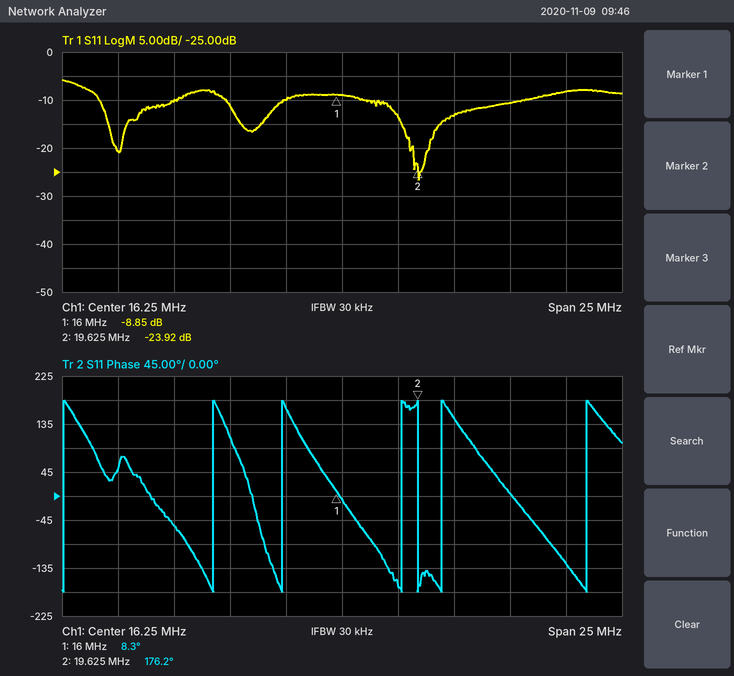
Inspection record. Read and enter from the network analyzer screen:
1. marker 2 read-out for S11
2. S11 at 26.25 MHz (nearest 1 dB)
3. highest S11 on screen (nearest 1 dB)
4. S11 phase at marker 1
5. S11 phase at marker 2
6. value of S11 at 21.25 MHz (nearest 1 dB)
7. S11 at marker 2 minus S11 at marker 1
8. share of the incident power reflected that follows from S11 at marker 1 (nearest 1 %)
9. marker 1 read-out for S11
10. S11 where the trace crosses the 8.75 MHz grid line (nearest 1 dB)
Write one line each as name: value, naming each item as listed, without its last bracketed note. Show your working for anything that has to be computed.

marker 2 read-out for S11: -23.92 dB
S11 at 26.25 MHz: -8 dB
highest S11 on screen: -6 dB
S11 phase at marker 1: 8.3°
S11 phase at marker 2: 176.2°
value of S11 at 21.25 MHz: -13 dB
S11 at marker 2 minus S11 at marker 1: -23.92 − (-8.85) = -15.07 dB
share of the incident power reflected that follows from S11 at marker 1: 10^(-8.85/10) ≈ 13 %
marker 1 read-out for S11: -8.85 dB
S11 where the trace crosses the 8.75 MHz grid line: -10 dB
